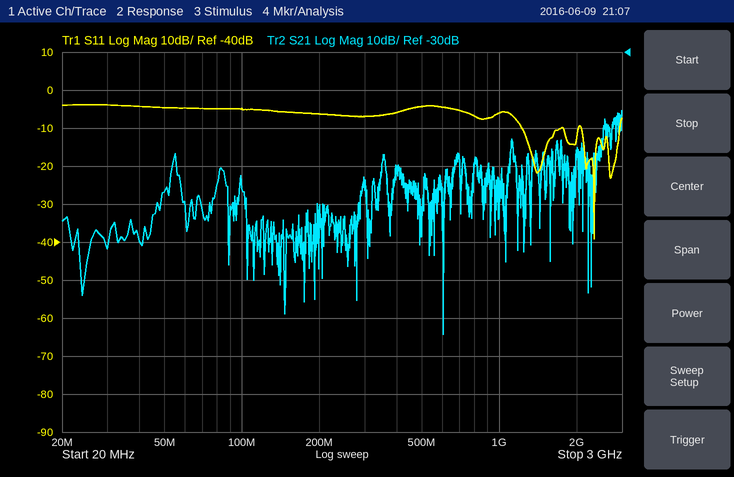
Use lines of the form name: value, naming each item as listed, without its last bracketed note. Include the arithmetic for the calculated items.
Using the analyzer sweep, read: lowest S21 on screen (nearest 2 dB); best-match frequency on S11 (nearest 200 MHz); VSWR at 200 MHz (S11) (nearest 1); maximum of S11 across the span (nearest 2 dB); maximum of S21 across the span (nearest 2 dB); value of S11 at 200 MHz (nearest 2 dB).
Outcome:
lowest S21 on screen: -104 dB
best-match frequency on S11: 2.4 GHz
VSWR at 200 MHz (S11): |Γ| = 10^(-6/20) = 0.5012; VSWR = (1 + 0.5012)/(1 − 0.5012) ≈ 3
maximum of S11 across the span: -4 dB
maximum of S21 across the span: -46 dB
value of S11 at 200 MHz: -6 dB
